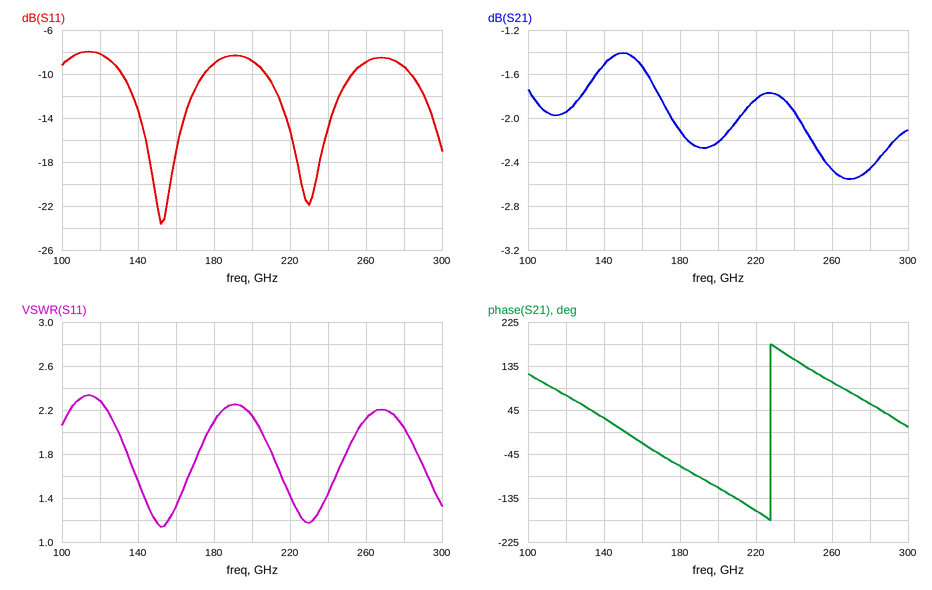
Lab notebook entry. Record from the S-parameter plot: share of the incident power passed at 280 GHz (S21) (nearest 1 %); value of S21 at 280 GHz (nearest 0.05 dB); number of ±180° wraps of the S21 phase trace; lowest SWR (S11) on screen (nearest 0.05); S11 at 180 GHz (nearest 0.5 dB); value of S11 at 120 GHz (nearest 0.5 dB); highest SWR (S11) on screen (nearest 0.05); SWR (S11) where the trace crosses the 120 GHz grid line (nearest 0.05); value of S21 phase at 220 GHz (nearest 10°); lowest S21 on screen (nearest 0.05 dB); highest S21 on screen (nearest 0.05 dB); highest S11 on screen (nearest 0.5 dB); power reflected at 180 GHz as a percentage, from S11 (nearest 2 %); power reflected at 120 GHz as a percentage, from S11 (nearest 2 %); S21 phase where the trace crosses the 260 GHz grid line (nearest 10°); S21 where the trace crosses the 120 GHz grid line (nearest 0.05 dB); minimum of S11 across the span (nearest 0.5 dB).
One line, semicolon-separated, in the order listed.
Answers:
57 %; -2.45 dB; 1; 1.15; -9.0 dB; -8.0 dB; 2.35; 2.30; -160°; -2.55 dB; -1.40 dB; -8.0 dB; 12 %; 16 %; 100°; -1.95 dB; -23.5 dB
